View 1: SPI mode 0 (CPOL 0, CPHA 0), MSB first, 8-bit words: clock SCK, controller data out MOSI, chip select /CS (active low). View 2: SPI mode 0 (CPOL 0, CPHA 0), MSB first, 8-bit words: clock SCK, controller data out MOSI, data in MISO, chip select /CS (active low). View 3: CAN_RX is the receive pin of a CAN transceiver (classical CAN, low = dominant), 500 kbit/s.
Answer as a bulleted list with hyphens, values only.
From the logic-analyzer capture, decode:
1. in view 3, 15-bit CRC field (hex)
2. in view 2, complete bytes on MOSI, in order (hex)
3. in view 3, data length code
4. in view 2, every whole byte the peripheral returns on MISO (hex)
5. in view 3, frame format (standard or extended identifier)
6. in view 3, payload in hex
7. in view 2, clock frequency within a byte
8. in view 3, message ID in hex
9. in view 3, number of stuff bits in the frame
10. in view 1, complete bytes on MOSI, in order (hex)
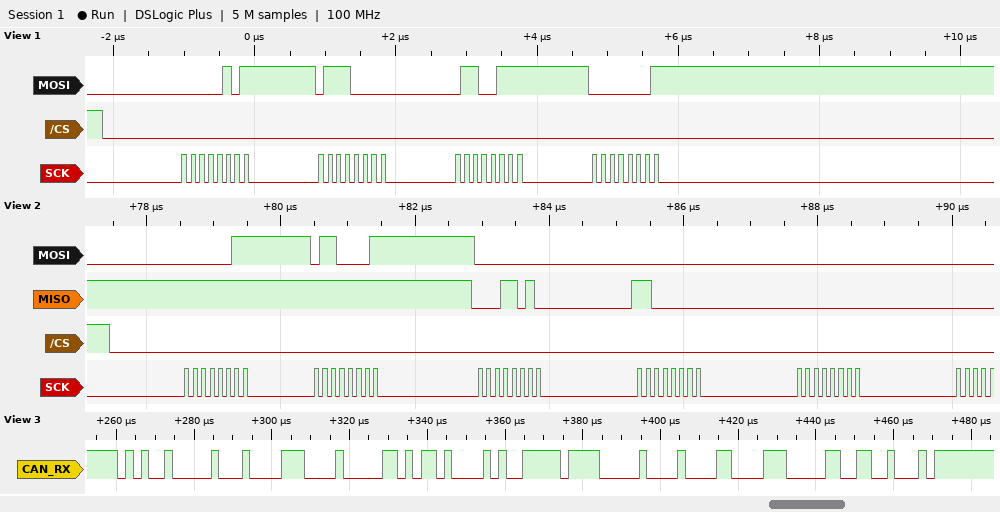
- 0x04C8
- 03 61 00 00 00
- 8
- FF FF 1A C0 00
- standard
- 70 82 B4 29 FF 00 43 0E
- 8 MHz
- 0x520
- 5
- 05 70 67 01
